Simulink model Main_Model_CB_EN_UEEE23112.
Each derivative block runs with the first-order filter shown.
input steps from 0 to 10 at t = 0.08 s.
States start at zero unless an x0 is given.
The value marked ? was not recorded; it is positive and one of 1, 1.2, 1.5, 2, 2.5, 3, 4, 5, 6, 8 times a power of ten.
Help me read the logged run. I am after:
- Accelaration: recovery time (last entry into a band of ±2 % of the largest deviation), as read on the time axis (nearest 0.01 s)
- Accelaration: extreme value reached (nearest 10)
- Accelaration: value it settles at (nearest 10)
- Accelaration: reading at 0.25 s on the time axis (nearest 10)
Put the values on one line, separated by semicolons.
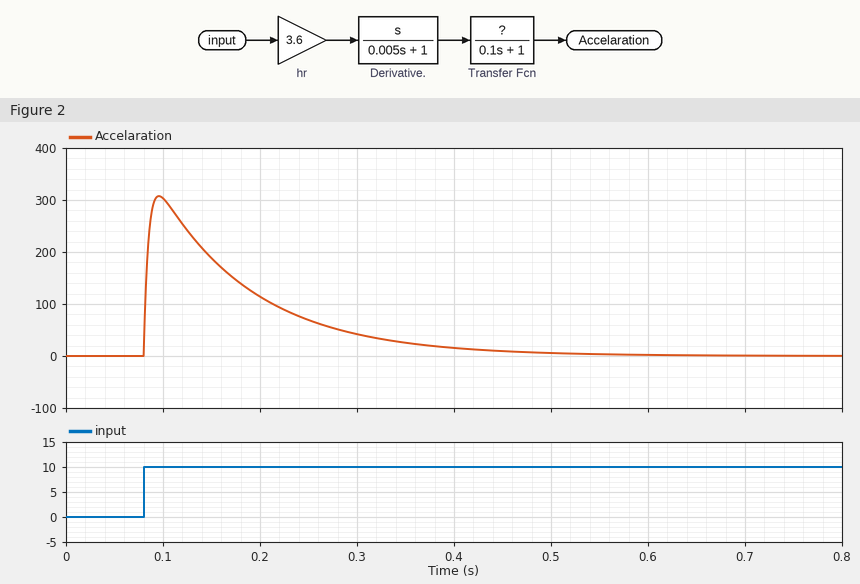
0.49 s; 310; 0; 70
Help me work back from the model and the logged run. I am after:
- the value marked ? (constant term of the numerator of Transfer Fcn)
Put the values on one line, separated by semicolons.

1
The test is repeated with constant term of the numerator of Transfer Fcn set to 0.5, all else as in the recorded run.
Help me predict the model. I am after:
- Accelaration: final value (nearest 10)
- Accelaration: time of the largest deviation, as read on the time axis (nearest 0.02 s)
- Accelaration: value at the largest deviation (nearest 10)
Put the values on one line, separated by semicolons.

0; 0.10 s; 150
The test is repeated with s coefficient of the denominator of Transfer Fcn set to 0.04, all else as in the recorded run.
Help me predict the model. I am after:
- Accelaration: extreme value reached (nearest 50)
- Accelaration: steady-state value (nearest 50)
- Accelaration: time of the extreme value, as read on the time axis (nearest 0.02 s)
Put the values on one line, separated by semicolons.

650; 0; 0.10 s
